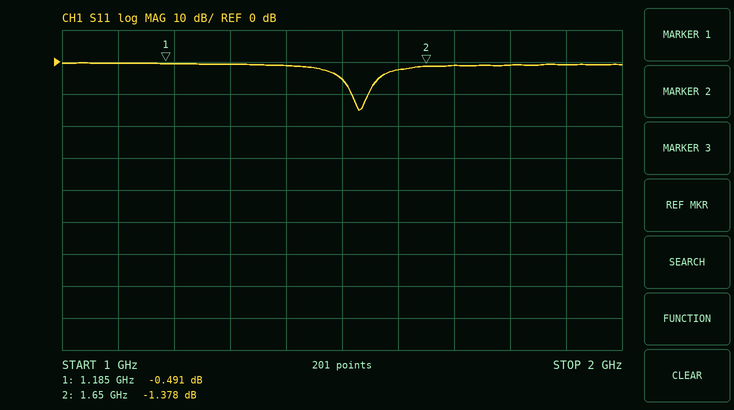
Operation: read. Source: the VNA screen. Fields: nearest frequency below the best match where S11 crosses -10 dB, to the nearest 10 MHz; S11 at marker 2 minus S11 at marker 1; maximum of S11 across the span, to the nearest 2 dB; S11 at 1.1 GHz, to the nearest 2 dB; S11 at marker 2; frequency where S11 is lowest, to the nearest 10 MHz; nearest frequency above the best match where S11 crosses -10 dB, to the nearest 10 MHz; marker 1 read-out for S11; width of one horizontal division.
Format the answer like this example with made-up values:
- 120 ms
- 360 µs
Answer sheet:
- 1.52 GHz
- -0.887 dB
- 0 dB
- 0 dB
- -1.378 dB
- 1.53 GHz
- 1.55 GHz
- -0.491 dB
- 100 MHz
